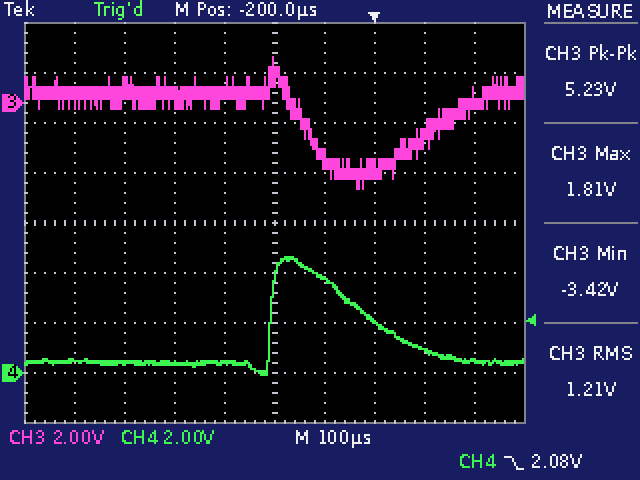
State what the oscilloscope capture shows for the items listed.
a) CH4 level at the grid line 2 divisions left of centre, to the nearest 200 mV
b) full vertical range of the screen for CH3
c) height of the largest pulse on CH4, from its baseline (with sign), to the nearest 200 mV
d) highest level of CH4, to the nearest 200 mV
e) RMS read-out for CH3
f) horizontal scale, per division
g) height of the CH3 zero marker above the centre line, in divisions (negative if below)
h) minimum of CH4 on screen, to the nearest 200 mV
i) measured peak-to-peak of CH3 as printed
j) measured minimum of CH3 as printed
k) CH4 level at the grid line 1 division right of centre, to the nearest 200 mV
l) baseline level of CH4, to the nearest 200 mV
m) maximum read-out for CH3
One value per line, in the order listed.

400 mV
16 V
+4.2 V
4.6 V
1.21 V
100 µs
+2.4 div
0.0 V
5.23 V
-3.42 V
3.8 V
400 mV
1.81 V
